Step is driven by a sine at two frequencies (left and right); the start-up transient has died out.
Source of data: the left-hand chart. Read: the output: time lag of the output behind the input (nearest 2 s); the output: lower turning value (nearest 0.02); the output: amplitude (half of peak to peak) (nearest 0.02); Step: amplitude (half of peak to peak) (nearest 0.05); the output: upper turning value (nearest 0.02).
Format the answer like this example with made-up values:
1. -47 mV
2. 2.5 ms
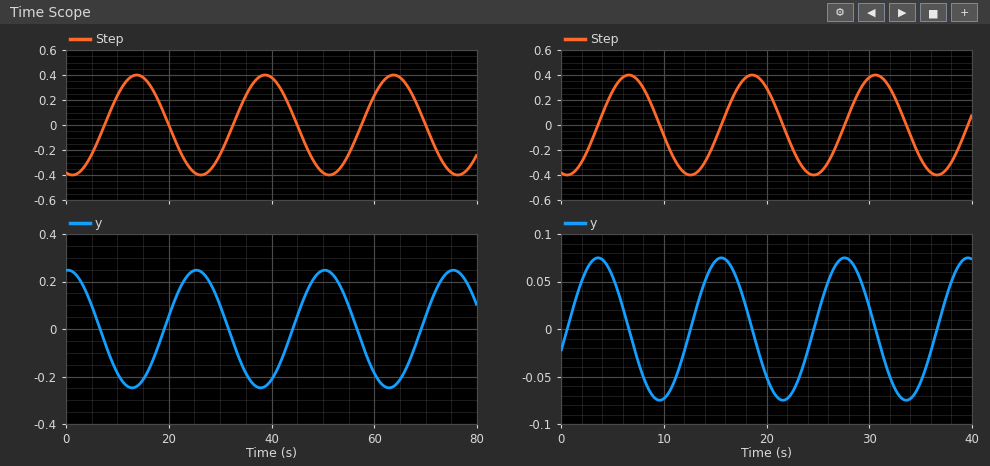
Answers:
1. 12 s
2. -0.24
3. 0.24
4. 0.40
5. 0.24
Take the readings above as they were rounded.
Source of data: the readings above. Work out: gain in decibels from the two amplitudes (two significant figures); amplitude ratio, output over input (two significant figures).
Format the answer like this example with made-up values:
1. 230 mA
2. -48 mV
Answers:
1. -4.4 dB
2. 0.60
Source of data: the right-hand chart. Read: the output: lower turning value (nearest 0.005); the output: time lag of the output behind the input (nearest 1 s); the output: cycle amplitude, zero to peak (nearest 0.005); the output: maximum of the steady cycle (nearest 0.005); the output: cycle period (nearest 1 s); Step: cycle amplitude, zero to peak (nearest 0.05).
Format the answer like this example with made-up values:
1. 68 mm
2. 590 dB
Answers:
1. -0.075
2. 9 s
3. 0.075
4. 0.075
5. 12 s
6. 0.40
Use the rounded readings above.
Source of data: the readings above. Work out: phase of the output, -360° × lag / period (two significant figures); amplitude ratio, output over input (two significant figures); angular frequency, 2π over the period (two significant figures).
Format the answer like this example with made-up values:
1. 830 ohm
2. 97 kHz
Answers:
1. -270°
2. 0.19
3. 0.52 rad/s
